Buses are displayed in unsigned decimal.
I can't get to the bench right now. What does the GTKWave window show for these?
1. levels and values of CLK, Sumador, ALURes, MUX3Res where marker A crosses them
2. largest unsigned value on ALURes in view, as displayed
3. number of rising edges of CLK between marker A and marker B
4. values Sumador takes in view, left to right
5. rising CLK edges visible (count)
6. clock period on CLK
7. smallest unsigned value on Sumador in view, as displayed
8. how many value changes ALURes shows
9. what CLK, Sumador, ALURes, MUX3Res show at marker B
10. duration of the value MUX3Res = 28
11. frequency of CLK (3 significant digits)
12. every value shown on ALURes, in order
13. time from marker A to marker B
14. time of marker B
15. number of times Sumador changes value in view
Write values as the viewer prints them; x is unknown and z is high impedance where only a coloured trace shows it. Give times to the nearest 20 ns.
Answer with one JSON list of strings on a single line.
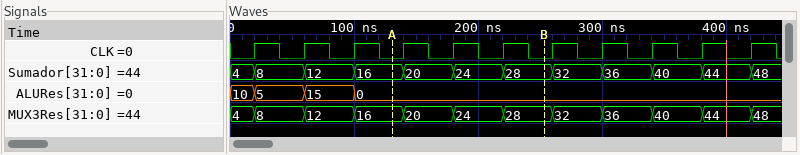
["CLK=0, Sumador=16, ALURes=0, MUX3Res=16", "15", "3", "4, 8, 12, 16, 20, 24, 28, 32, 36, 40, 44, 48", "11", "40 ns", "4", "3", "CLK=0, Sumador=28, ALURes=0, MUX3Res=28", "40 ns", "25.0 MHz", "10, 5, 15, 0", "120 ns", "260 ns", "11"]
